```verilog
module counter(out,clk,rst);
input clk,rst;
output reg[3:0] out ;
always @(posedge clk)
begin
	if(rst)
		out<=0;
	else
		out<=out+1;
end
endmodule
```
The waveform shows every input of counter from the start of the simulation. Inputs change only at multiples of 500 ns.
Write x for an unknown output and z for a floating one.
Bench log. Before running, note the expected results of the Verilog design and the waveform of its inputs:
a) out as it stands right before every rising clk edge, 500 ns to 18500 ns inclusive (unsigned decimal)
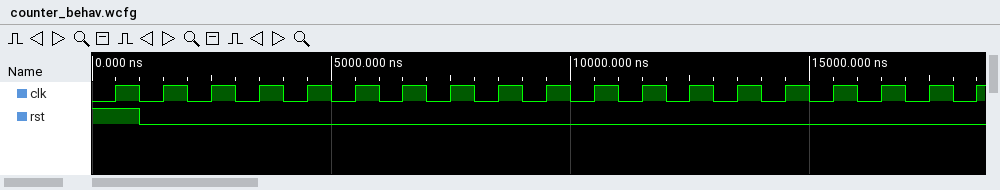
x, 0, 1, 2, 3, 4, 5, 6, 7, 8, 9, 10, 11, 12, 13, 14, 15, 0, 1
